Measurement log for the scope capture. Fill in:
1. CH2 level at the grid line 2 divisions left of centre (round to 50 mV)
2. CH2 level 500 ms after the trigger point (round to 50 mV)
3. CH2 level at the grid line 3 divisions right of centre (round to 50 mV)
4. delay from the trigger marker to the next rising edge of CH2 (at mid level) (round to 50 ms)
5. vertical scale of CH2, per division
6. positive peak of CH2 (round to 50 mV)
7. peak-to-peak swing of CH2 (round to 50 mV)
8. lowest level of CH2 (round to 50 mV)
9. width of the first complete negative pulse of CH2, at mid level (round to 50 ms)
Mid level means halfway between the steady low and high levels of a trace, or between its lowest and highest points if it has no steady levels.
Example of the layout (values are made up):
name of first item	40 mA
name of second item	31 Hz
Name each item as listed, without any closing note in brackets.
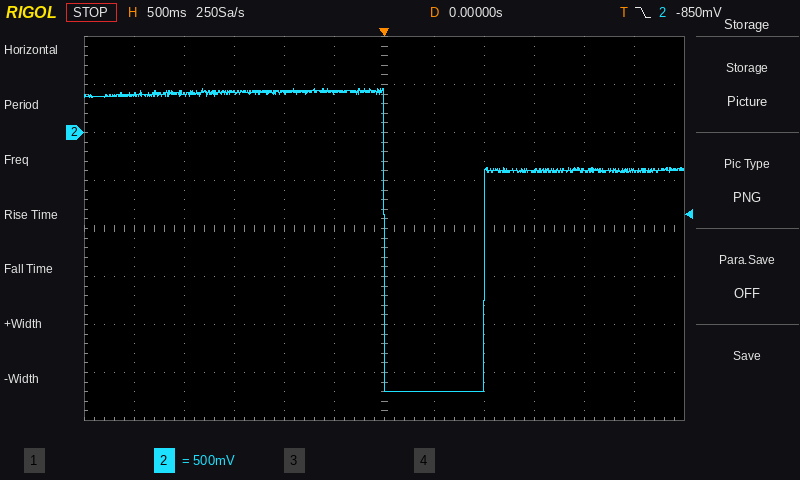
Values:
CH2 level at the grid line 2 divisions left of centre	400 mV
CH2 level 500 ms after the trigger point	-2.70 V
CH2 level at the grid line 3 divisions right of centre	-400 mV
delay from the trigger marker to the next rising edge of CH2 (at mid level)	1.00 s
vertical scale of CH2, per division	500 mV
positive peak of CH2	450 mV
peak-to-peak swing of CH2	3.15 V
lowest level of CH2	-2.70 V
width of the first complete negative pulse of CH2, at mid level	1.00 s
